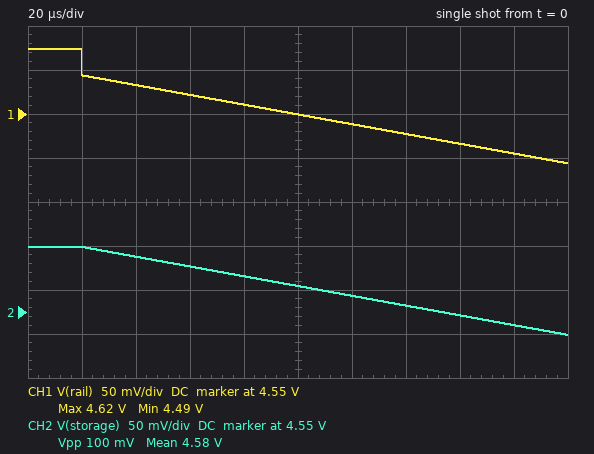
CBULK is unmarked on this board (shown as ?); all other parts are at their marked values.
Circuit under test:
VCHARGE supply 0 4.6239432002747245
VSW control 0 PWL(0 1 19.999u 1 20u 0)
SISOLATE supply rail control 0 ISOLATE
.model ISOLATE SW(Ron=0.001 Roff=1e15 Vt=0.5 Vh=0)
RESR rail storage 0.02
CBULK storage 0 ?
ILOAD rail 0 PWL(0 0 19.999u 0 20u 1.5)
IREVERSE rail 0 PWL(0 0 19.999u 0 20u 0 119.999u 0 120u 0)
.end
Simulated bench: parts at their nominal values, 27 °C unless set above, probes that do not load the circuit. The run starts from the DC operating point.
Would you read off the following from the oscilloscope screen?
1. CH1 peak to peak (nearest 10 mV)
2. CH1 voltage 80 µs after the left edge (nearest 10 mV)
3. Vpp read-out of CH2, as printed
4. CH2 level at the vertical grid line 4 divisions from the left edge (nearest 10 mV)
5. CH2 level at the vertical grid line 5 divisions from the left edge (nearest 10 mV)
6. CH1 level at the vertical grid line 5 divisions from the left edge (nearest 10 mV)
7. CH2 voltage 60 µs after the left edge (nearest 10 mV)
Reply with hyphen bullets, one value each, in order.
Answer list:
- 130 mV
- 4.56 V
- 100 mV
- 4.59 V
- 4.58 V
- 4.55 V
- 4.60 V
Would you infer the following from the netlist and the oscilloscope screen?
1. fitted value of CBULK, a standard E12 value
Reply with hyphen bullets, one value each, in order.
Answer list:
- 2.7 mF
